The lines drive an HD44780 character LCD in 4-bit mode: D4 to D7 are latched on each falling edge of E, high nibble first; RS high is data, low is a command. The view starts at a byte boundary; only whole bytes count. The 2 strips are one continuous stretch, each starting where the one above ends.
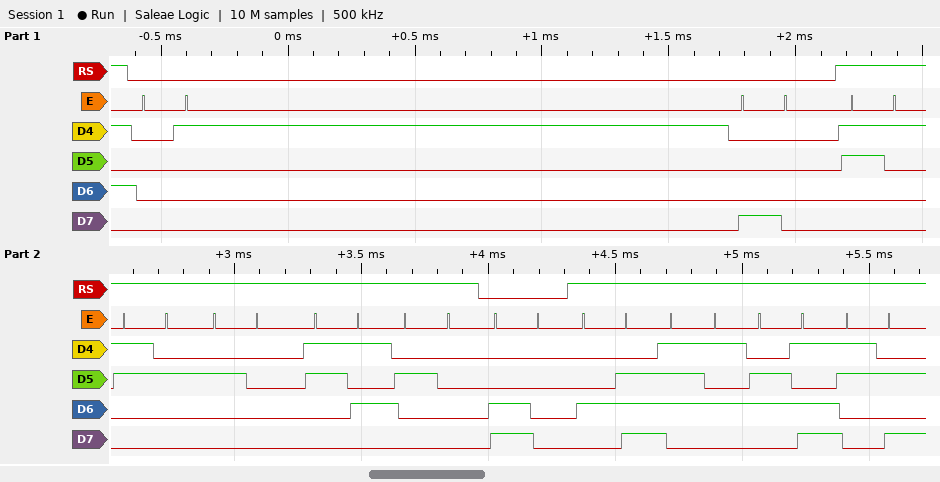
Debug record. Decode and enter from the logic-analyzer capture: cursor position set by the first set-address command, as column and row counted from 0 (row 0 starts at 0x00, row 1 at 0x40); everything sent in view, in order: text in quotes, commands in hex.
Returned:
column 0, row 0
0x01 0x80 "12 5 " 0xC0 "Num:"
